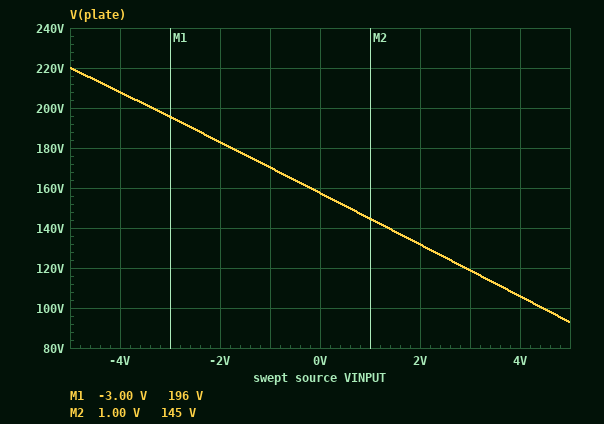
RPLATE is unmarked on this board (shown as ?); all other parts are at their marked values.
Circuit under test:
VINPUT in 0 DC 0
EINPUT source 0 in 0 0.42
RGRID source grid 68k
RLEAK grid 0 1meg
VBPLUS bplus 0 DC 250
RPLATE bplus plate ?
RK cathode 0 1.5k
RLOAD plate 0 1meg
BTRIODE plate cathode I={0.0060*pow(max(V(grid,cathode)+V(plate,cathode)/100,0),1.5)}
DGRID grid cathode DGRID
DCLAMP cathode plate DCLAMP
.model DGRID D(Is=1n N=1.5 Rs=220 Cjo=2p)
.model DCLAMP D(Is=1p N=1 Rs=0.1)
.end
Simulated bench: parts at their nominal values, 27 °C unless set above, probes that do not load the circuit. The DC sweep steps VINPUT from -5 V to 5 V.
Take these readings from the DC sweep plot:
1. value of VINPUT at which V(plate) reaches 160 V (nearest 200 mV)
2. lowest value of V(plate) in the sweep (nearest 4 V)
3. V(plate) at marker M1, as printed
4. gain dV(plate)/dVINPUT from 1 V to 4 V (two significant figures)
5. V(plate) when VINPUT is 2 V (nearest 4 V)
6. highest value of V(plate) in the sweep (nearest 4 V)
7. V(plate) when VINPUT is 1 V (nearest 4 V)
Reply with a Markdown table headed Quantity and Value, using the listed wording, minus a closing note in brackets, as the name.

| Quantity | Value |
|---|---|
| value of VINPUT at which V(plate) reaches 160 V | -200 mV |
| lowest value of V(plate) in the sweep | 92 V |
| V(plate) at marker M1, as printed | 196 V |
| gain dV(plate)/dVINPUT from 1 V to 4 V | -13 V/V |
| V(plate) when VINPUT is 2 V | 132 V |
| highest value of V(plate) in the sweep | 220 V |
| V(plate) when VINPUT is 1 V | 144 V |
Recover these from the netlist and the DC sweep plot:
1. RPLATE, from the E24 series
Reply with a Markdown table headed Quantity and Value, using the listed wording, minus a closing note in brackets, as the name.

| Quantity | Value |
|---|---|
| RPLATE, from the E24 series | 91 kΩ |
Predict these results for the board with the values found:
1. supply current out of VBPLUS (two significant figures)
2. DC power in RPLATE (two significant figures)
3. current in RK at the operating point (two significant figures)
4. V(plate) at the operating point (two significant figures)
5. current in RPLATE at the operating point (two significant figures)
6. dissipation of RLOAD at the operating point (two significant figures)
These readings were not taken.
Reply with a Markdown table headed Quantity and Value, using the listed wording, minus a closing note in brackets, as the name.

| Quantity | Value |
|---|---|
| supply current out of VBPLUS | 1.0 mA |
| DC power in RPLATE | 94 mW |
| current in RK at the operating point | 860 µA |
| V(plate) at the operating point | 160 V |
| current in RPLATE at the operating point | 1.0 mA |
| dissipation of RLOAD at the operating point | 25 mW |
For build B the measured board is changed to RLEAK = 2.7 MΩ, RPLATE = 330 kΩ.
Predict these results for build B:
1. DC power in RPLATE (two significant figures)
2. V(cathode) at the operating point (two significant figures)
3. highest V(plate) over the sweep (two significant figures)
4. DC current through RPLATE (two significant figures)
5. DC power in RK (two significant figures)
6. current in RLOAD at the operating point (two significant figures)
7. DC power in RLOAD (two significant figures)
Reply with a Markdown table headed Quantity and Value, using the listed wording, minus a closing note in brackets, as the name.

| Quantity | Value |
|---|---|
| DC power in RPLATE | 86 mW |
| V(cathode) at the operating point | 640 mV |
| highest V(plate) over the sweep | 190 V |
| DC current through RPLATE | 510 µA |
| DC power in RK | 270 µW |
| current in RLOAD at the operating point | 82 µA |
| DC power in RLOAD | 6.7 mW |
